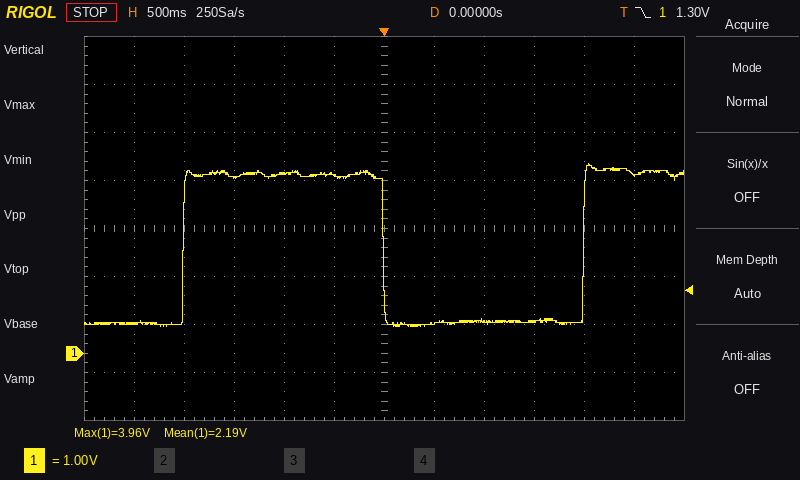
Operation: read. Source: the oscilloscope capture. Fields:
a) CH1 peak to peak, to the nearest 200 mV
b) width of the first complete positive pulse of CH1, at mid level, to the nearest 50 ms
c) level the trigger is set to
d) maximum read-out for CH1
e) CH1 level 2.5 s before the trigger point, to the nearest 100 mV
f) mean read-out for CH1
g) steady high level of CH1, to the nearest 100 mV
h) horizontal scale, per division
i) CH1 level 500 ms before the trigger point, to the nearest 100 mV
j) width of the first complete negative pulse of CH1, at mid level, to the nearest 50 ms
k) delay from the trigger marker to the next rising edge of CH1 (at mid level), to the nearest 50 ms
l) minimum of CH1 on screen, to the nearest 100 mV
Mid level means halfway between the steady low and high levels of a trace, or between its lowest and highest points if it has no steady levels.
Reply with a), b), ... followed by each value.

a) 3.4 V
b) 2.00 s
c) 1.30 V
d) 3.96 V
e) 600 mV
f) 2.19 V
g) 3.7 V
h) 500 ms
i) 3.7 V
j) 2.00 s
k) 2.00 s
l) 600 mV
